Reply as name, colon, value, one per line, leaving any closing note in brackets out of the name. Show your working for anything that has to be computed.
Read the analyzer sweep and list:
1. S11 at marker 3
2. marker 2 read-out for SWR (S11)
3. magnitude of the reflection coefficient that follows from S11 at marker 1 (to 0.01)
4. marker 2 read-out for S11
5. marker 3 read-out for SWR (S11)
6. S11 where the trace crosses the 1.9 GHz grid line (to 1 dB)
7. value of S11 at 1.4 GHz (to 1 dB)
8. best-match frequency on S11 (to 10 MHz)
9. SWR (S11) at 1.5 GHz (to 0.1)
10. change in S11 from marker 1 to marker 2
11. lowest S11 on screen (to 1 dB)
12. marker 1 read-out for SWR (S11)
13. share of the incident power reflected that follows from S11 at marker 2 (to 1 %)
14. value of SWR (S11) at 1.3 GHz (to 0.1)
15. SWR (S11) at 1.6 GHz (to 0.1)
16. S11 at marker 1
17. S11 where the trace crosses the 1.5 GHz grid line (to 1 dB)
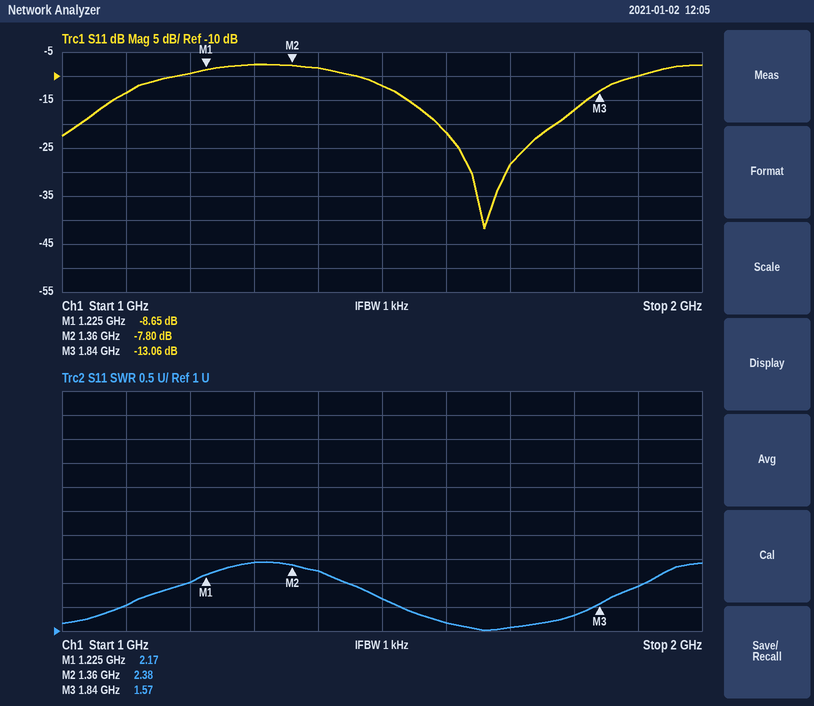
S11 at marker 3: -13.06 dB
marker 2 read-out for SWR: 2.38
magnitude of the reflection coefficient that follows from S11 at marker 1: 10^(-8.65/20) ≈ 0.37
marker 2 read-out for S11: -7.80 dB
marker 3 read-out for SWR: 1.57
S11 where the trace crosses the 1.9 GHz grid line: -10 dB
value of S11 at 1.4 GHz: -8 dB
best-match frequency on S11: 1.66 GHz
SWR (S11) at 1.5 GHz: 1.7
change in S11 from marker 1 to marker 2: -7.8 − (-8.65) = 0.85 dB
lowest S11 on screen: -42 dB
marker 1 read-out for SWR: 2.17
share of the incident power reflected that follows from S11 at marker 2: 10^(-7.8/10) ≈ 17 %
value of SWR (S11) at 1.3 GHz: 2.4
SWR (S11) at 1.6 GHz: 1.2
S11 at marker 1: -8.65 dB
S11 where the trace crosses the 1.5 GHz grid line: -12 dB
